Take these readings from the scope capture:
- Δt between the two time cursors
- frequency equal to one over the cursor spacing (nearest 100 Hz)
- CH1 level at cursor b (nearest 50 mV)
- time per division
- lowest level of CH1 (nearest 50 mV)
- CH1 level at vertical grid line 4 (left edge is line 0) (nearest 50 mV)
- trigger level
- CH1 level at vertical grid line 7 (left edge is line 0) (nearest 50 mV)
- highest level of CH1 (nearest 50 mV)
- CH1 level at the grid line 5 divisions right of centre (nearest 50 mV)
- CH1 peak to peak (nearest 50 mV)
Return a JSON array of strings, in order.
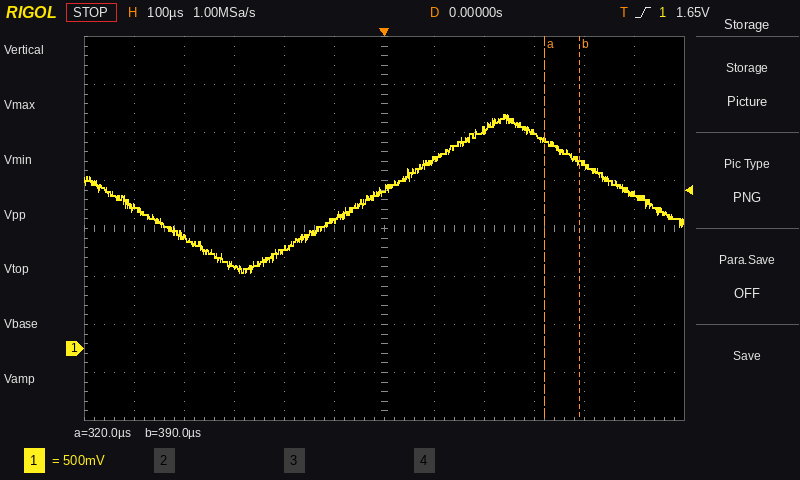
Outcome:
["70 µs", "14.3 kHz", "1.95 V", "100 µs", "800 mV", "1.05 V", "1.65 V", "1.95 V", "2.45 V", "1.60 V", "1.65 V"]
